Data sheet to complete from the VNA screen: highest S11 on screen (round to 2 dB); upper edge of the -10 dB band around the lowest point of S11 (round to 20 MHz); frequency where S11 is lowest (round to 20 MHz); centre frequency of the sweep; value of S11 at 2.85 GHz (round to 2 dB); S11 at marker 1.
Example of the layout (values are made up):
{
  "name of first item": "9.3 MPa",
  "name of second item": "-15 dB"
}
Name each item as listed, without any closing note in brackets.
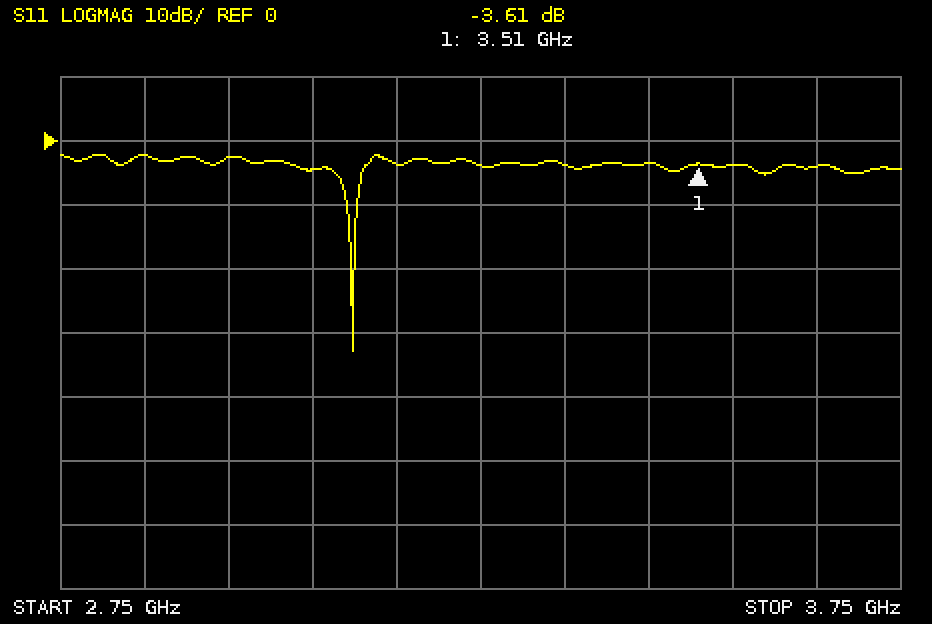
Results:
{
  "highest S11 on screen": "-2 dB",
  "upper edge of the -10 dB band around the lowest point of S11": "3.10 GHz",
  "frequency where S11 is lowest": "3.10 GHz",
  "centre frequency of the sweep": "3.25 GHz",
  "value of S11 at 2.85 GHz": "-2 dB",
  "S11 at marker 1": "-3.61 dB"
}
